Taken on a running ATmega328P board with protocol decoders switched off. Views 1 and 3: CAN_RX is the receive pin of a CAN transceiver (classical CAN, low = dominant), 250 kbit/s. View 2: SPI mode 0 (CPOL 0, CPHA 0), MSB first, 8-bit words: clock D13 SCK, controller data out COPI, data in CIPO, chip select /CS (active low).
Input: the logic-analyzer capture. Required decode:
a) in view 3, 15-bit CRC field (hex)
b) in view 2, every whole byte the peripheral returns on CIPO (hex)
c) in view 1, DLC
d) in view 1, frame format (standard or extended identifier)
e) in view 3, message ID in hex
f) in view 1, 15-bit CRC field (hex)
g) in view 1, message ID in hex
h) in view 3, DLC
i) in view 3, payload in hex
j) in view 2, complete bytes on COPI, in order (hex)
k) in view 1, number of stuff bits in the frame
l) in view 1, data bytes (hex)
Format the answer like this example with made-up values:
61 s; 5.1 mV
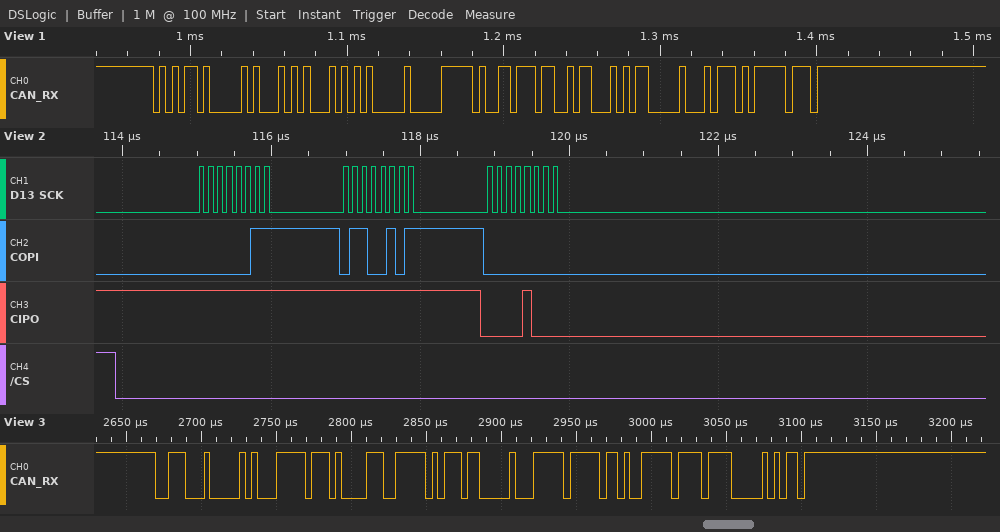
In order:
0x5E05; 0xFF 0xFF 0x08; 8; standard; 0x388; 0x5D7F; 0x568; 8; FF 43 9F BB 00 FF F4 FF; 0x03 0x65 0x00; 6; A8 AA 00 7C DD 96 2B 00
